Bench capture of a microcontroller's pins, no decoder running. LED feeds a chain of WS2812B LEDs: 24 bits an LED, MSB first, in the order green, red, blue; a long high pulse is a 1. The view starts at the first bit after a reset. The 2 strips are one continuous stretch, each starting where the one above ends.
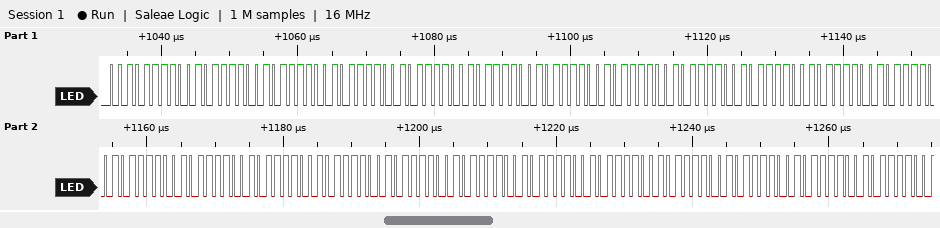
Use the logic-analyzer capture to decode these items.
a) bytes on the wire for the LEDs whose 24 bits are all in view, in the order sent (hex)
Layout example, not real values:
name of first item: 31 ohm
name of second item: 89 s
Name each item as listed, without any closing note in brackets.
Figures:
bytes on the wire for the LEDs whose 24 bits are all in view, in the order sent: 2F 2F 2F 2F 2F 2F 2F 2F 2F 2F 2F 2F 2F 2F 2F 2F 2F 2F 2F 2F 2F 2F 2F 2F
